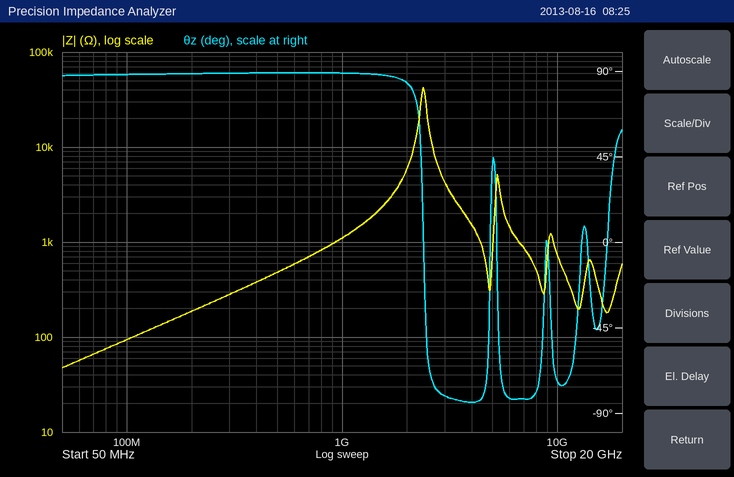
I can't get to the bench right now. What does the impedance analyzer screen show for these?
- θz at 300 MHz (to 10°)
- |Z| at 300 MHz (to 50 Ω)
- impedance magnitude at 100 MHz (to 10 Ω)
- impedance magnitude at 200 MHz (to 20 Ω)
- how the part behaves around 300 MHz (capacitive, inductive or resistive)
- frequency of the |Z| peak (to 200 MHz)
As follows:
90°
300 Ω
90 Ω
180 Ω
inductive
2.4 GHz
